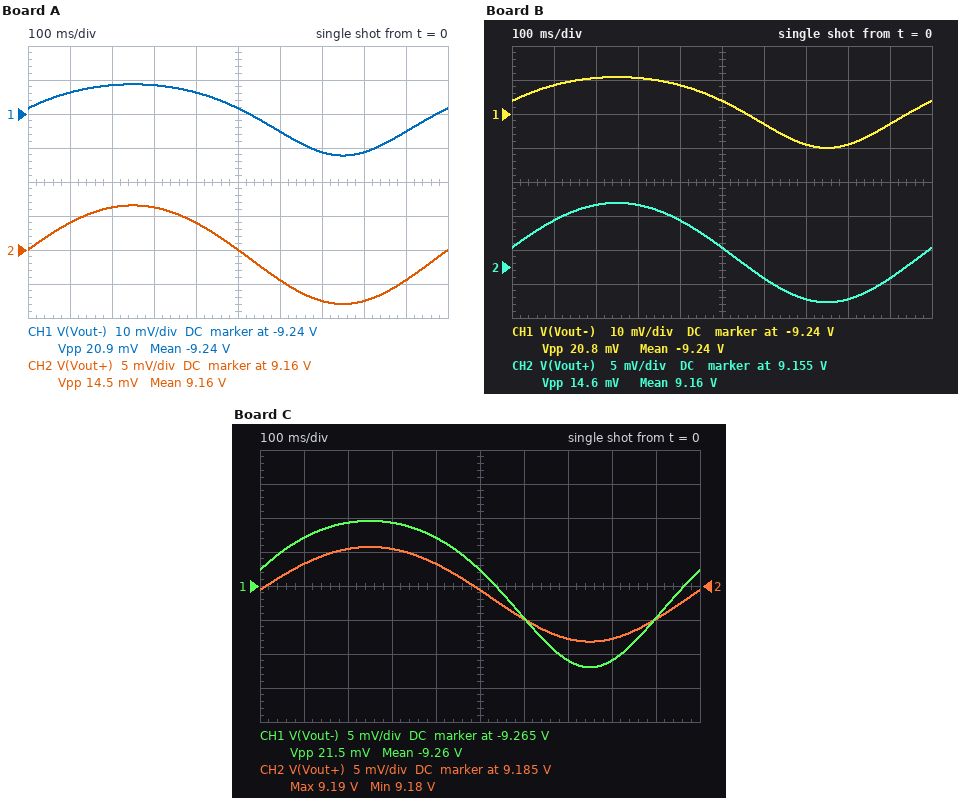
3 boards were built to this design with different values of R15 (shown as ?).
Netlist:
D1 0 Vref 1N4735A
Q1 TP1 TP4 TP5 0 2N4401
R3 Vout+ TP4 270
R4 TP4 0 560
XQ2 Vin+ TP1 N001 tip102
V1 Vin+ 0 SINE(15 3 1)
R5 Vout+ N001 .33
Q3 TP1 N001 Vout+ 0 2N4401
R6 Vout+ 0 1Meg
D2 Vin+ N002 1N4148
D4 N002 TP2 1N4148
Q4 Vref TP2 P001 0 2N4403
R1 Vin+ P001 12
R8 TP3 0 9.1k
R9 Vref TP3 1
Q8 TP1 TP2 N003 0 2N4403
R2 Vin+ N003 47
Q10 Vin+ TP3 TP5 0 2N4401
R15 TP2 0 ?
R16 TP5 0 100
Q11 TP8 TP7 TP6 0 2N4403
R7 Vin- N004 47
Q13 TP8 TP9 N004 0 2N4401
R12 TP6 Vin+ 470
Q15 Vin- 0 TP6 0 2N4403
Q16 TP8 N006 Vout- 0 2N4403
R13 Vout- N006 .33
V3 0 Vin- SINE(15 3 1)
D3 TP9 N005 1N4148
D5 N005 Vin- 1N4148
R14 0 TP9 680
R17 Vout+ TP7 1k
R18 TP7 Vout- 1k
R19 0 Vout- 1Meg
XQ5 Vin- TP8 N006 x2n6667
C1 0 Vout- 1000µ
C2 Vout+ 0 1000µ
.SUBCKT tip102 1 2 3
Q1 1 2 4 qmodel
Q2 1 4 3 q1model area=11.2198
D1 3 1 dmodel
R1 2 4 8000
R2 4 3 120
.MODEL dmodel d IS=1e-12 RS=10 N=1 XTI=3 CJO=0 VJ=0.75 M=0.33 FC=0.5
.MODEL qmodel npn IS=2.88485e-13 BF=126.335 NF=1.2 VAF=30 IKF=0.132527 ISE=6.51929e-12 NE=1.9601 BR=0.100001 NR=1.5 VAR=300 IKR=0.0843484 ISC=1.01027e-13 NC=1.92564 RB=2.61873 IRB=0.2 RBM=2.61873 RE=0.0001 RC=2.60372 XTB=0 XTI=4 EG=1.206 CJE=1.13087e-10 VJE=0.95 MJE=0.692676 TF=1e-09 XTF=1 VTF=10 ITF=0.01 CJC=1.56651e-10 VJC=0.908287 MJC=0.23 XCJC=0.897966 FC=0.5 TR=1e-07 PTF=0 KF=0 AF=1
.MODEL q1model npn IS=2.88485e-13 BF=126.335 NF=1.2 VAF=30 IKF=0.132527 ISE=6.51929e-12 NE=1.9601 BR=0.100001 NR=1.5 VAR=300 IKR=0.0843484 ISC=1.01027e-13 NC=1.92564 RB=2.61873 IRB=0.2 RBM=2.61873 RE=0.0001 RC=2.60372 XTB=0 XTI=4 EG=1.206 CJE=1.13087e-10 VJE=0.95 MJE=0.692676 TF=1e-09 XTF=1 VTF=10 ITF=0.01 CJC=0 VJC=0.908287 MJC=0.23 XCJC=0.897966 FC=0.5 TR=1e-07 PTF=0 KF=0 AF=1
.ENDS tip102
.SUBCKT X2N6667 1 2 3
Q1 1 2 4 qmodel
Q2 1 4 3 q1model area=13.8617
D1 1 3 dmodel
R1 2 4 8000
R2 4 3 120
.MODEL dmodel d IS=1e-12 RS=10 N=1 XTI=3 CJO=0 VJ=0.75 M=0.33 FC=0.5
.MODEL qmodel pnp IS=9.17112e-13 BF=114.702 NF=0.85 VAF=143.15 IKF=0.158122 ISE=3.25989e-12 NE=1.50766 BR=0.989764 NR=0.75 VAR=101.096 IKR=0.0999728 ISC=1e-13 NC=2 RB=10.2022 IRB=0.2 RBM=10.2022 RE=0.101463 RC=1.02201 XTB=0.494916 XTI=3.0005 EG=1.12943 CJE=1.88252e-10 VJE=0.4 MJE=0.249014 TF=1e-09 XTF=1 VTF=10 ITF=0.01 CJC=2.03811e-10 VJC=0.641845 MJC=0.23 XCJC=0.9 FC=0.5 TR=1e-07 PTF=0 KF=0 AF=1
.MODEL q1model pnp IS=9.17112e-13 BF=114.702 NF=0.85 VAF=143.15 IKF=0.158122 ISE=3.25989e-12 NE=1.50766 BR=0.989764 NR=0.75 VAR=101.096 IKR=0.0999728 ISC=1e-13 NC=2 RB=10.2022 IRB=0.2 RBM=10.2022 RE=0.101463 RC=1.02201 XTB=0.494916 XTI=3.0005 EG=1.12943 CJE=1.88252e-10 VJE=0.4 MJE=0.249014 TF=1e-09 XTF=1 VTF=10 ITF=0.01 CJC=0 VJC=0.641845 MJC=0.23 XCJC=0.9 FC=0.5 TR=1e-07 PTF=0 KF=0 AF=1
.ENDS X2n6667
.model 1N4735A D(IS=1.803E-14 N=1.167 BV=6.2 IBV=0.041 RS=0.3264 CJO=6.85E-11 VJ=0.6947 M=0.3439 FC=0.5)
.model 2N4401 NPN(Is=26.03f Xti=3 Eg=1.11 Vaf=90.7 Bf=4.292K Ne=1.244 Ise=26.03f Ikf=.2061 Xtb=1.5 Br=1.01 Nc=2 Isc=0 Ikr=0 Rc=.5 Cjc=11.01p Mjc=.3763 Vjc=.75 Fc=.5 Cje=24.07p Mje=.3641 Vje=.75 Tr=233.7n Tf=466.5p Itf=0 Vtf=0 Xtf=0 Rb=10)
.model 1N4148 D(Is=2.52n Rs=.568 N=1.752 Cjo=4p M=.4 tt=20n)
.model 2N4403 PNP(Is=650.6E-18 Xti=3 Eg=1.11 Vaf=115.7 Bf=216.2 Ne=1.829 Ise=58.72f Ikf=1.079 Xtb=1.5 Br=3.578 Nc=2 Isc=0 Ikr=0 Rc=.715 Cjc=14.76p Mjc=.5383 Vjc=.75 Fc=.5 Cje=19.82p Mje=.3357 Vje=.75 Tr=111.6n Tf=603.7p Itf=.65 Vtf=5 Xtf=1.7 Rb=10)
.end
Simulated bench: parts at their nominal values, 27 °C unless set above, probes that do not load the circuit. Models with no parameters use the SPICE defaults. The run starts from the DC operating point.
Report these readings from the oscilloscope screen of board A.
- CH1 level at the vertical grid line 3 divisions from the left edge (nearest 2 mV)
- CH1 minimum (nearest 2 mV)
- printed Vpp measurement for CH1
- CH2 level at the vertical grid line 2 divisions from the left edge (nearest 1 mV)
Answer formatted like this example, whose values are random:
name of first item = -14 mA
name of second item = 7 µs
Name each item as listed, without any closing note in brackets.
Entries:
CH1 level at the vertical grid line 3 divisions from the left edge = -9.232 V
CH1 minimum = -9.252 V
printed Vpp measurement for CH1 = 20.9 mV
CH2 level at the vertical grid line 2 divisions from the left edge = 9.166 V
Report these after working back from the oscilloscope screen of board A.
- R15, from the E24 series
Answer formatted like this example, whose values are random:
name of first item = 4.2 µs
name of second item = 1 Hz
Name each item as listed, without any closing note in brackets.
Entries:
R15, from the E24 series = 3.3 kΩ
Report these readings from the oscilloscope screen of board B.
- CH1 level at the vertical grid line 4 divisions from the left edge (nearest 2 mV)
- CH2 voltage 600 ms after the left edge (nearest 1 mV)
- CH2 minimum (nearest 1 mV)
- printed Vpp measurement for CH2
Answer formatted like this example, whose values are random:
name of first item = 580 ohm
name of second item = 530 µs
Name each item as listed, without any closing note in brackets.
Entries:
CH1 level at the vertical grid line 4 divisions from the left edge = -9.232 V
CH2 voltage 600 ms after the left edge = 9.153 V
CH2 minimum = 9.150 V
printed Vpp measurement for CH2 = 14.6 mV
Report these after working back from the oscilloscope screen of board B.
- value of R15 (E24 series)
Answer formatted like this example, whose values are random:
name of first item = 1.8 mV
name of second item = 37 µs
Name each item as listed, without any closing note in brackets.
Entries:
value of R15 = 3.6 kΩ
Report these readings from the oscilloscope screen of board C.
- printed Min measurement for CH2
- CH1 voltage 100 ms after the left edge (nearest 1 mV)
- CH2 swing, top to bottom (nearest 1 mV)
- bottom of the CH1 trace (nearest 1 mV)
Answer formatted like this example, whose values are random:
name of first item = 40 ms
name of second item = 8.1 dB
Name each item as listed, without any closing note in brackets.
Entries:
printed Min measurement for CH2 = 9.18 V
CH1 voltage 100 ms after the left edge = -9.258 V
CH2 swing, top to bottom = 14 mV
bottom of the CH1 trace = -9.277 V
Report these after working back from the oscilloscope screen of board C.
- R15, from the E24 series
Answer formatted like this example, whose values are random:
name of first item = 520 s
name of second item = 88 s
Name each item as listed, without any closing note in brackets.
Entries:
R15, from the E24 series = 1.2 kΩ
